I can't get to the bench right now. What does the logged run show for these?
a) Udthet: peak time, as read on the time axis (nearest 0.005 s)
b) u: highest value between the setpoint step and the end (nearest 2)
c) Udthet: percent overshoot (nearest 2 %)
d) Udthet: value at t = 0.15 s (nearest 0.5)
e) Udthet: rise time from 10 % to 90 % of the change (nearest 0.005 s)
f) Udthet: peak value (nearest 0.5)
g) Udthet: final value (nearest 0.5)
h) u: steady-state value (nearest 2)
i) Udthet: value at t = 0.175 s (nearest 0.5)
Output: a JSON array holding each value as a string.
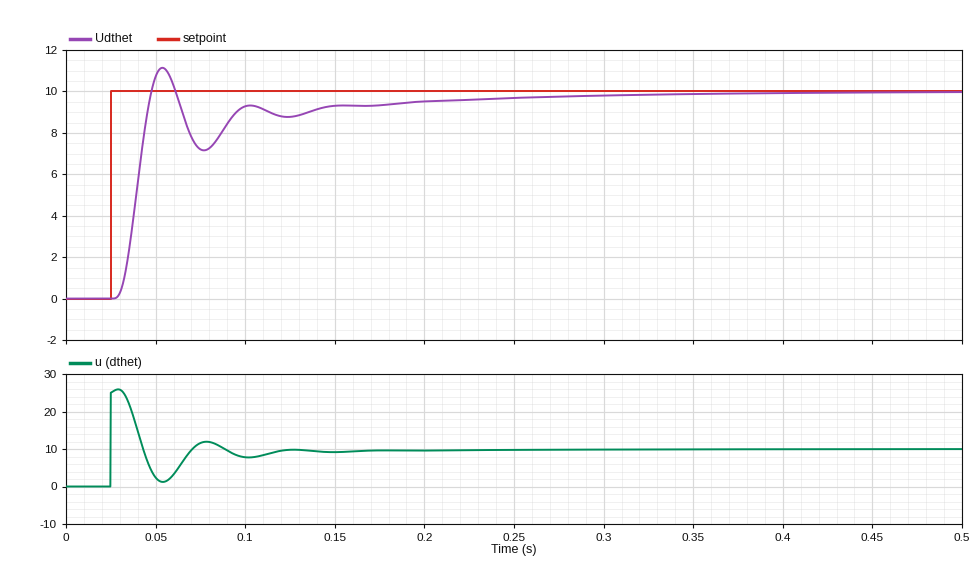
["0.055 s", "26", "12 %", "9.5", "0.015 s", "11.0", "10.0", "10", "9.5"]
